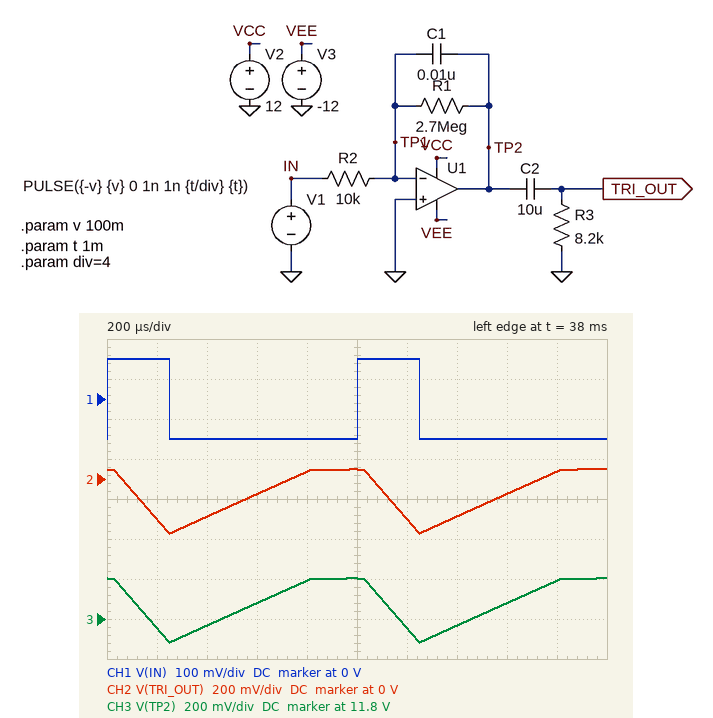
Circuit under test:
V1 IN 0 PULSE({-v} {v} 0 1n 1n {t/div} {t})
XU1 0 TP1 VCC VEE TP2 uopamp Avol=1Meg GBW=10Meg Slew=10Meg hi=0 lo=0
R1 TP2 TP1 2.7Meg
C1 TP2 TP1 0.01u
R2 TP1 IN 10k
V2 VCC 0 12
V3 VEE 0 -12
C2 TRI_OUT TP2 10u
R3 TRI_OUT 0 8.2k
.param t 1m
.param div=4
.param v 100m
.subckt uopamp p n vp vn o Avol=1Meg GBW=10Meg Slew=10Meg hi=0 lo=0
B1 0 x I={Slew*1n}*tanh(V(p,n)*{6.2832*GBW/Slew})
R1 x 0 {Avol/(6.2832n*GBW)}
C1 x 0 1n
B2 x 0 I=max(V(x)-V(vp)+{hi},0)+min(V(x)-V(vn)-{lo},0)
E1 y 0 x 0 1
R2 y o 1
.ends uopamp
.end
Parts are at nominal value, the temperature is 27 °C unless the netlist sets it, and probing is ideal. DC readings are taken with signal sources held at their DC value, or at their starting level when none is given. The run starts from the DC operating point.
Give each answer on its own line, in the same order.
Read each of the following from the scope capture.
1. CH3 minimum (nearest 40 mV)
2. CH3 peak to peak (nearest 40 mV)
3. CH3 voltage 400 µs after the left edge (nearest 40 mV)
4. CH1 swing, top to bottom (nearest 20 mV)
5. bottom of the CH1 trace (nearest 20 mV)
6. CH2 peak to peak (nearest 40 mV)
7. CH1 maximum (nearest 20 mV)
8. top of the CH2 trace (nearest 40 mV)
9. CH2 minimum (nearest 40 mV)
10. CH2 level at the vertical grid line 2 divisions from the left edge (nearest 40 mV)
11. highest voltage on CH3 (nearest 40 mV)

11.68 V
320 mV
11.76 V
200 mV
-100 mV
320 mV
100 mV
40 mV
-280 mV
-200 mV
12.00 V
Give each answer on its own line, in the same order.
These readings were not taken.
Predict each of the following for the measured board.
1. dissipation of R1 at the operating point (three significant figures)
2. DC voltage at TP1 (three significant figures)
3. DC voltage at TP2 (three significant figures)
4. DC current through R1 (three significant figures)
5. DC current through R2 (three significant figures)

53.9 µW
-55.3 mV
12.0 V
4.47 µA
4.47 µA
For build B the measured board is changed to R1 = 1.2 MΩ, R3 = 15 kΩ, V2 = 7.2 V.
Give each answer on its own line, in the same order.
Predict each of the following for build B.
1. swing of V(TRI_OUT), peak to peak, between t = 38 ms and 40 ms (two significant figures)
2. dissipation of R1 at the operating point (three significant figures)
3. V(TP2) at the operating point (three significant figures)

380 mV
43.7 µW
7.20 V
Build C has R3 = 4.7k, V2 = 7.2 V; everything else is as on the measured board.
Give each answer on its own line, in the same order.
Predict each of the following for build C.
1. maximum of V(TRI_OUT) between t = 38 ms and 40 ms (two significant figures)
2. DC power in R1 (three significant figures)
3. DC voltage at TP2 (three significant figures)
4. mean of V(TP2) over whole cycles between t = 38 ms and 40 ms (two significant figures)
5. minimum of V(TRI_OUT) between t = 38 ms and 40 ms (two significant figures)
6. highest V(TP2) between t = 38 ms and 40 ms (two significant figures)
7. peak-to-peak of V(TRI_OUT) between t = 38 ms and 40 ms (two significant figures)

42 mV
19.6 µW
7.20 V
7.1 V
-220 mV
7.2 V
260 mV
